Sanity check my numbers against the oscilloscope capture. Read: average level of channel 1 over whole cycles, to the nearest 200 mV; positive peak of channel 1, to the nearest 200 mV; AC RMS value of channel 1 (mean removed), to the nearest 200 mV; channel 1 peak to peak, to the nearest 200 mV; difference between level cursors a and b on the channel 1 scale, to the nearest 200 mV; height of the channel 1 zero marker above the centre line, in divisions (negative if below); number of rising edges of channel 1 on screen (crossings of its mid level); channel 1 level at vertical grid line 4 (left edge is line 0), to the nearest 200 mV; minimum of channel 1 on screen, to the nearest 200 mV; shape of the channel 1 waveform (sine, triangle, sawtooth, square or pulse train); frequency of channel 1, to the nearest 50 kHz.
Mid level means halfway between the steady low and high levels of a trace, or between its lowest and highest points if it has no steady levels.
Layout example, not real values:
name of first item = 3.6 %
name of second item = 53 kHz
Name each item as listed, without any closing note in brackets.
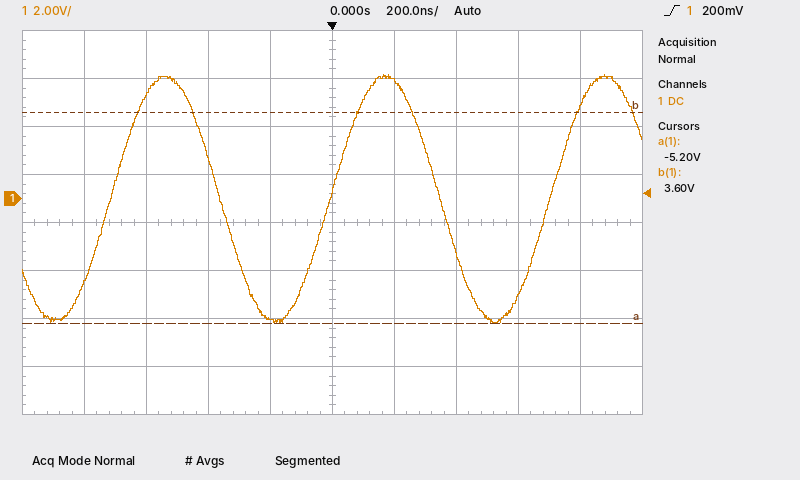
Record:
average level of channel 1 over whole cycles, to the nearest 200 mV = 0.0 V
positive peak of channel 1, to the nearest 200 mV = 5.2 V
AC RMS value of channel 1 (mean removed), to the nearest 200 mV = 3.6 V
channel 1 peak to peak, to the nearest 200 mV = 10.4 V
difference between level cursors a and b on the channel 1 scale, to the nearest 200 mV = 8.8 V
height of the channel 1 zero marker above the centre line, in divisions = +0.5 div
number of rising edges of channel 1 on screen = 3
channel 1 level at vertical grid line 4 (left edge is line 0), to the nearest 200 mV = -5.0 V
minimum of channel 1 on screen, to the nearest 200 mV = -5.2 V
shape of the channel 1 waveform = sine
frequency of channel 1, to the nearest 50 kHz = 1.40 MHz
